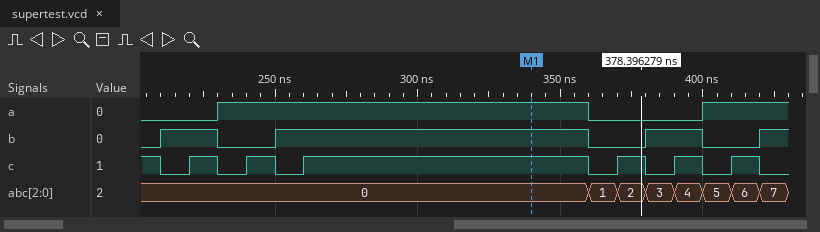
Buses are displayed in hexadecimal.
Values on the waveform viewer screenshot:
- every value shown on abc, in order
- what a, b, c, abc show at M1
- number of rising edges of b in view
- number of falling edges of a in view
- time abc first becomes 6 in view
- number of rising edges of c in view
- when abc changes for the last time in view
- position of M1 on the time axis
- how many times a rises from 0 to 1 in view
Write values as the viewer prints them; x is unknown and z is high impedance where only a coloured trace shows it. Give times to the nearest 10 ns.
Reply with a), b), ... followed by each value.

a) 0, 1, 2, 3, 4, 5, 6, 7
b) a=1, b=1, c=1, abc=0
c) 4
d) 1
e) 410 ns
f) 6
g) 420 ns
h) 340 ns
i) 2
